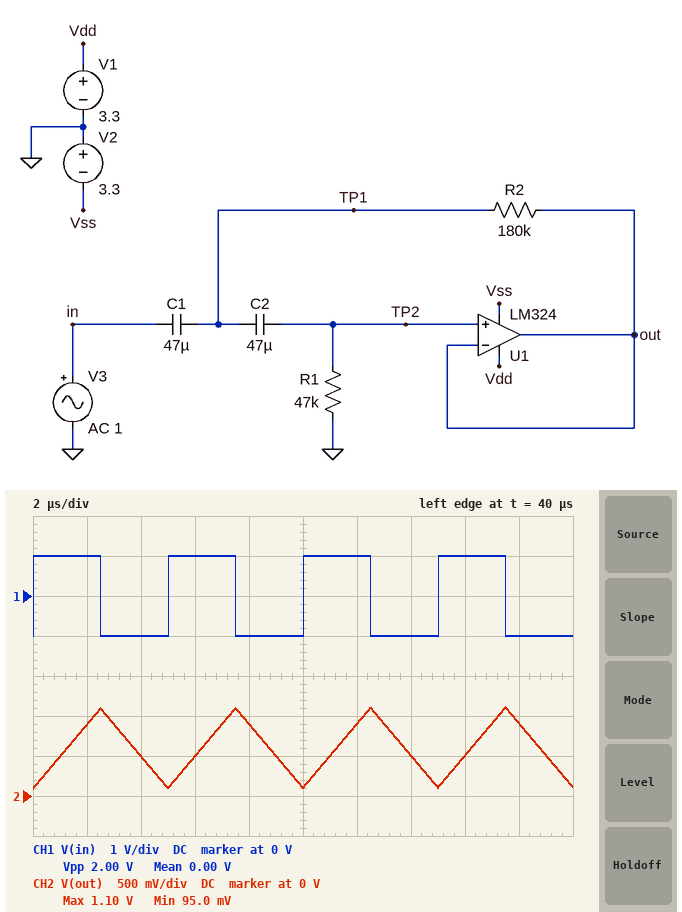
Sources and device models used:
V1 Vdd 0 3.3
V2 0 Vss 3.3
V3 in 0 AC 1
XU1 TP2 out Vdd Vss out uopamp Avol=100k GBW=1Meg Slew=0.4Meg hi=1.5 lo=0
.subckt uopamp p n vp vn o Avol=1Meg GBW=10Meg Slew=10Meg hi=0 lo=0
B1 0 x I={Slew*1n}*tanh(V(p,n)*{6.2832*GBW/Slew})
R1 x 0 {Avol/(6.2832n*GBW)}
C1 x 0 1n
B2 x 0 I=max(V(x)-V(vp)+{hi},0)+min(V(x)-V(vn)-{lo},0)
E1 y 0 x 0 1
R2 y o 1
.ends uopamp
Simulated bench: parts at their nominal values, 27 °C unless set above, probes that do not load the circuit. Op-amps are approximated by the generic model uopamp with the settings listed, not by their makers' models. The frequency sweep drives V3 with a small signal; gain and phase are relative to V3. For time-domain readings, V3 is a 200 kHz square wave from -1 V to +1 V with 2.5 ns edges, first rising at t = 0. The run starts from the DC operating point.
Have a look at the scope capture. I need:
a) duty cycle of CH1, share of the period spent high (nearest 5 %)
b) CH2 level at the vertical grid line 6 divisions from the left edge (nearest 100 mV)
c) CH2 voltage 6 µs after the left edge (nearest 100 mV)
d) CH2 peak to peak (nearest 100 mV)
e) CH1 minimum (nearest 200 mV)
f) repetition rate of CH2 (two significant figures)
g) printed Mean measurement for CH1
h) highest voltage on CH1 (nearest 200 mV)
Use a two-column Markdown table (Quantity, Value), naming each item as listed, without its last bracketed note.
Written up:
| Quantity | Value |
|---|---|
| duty cycle of CH1, share of the period spent high | 50 % |
| CH2 level at the vertical grid line 6 divisions from the left edge | 900 mV |
| CH2 voltage 6 µs after the left edge | 500 mV |
| CH2 peak to peak | 1.0 V |
| CH1 minimum | -1.0 V |
| repetition rate of CH2 | 200 kHz |
| printed Mean measurement for CH1 | 0.00 V |
| highest voltage on CH1 | 1.0 V |
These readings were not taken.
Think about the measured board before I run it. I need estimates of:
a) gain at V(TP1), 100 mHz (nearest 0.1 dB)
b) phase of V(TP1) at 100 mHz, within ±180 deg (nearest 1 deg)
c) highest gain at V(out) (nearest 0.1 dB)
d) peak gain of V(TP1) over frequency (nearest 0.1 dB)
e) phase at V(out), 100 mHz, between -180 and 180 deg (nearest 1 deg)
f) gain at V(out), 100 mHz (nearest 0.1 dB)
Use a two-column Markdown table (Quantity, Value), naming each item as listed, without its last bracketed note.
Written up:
| Quantity | Value |
|---|---|
| gain at V(TP1), 100 mHz | -2.7 dB |
| phase of V(TP1) at 100 mHz, within ±180 deg | 23 deg |
| highest gain at V(out) | 0 dB |
| peak gain of V(TP1) over frequency | 0 dB |
| phase at V(out), 100 mHz, between -180 and 180 deg | 59 deg |
| gain at V(out), 100 mHz | -4.5 dB |
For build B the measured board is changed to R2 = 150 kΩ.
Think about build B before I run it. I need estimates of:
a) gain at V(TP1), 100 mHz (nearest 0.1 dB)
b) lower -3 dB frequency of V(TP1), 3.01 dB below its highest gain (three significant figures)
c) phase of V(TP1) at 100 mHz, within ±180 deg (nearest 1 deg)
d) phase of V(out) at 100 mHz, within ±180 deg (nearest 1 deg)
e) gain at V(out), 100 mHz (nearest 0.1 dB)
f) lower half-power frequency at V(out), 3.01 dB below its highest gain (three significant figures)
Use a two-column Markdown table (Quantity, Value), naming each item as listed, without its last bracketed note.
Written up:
| Quantity | Value |
|---|---|
| gain at V(TP1), 100 mHz | -2.6 dB |
| lower -3 dB frequency of V(TP1), 3.01 dB below its highest gain | 86.5 mHz |
| phase of V(TP1) at 100 mHz, within ±180 deg | 24 deg |
| phase of V(out) at 100 mHz, within ±180 deg | 60 deg |
| gain at V(out), 100 mHz | -4.4 dB |
| lower half-power frequency at V(out), 3.01 dB below its highest gain | 133 mHz |
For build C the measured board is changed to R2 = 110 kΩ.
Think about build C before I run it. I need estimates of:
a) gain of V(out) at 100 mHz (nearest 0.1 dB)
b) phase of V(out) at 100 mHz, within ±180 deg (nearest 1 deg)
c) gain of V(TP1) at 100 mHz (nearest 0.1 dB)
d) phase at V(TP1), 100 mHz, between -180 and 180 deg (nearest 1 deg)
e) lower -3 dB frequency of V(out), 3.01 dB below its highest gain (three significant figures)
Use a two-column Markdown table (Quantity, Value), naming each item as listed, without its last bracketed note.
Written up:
| Quantity | Value |
|---|---|
| gain of V(out) at 100 mHz | -4.3 dB |
| phase of V(out) at 100 mHz, within ±180 deg | 62 deg |
| gain of V(TP1) at 100 mHz | -2.5 dB |
| phase at V(TP1), 100 mHz, between -180 and 180 deg | 26 deg |
| lower -3 dB frequency of V(out), 3.01 dB below its highest gain | 129 mHz |
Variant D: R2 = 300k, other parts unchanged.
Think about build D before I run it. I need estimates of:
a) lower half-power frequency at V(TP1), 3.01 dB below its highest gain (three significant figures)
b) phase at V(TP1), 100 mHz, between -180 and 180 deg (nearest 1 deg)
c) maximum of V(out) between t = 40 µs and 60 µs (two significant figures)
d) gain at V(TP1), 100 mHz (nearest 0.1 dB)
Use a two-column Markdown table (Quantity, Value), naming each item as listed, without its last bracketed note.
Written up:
| Quantity | Value |
|---|---|
| lower half-power frequency at V(TP1), 3.01 dB below its highest gain | 94.0 mHz |
| phase at V(TP1), 100 mHz, between -180 and 180 deg | 22 deg |
| maximum of V(out) between t = 40 µs and 60 µs | 1.1 V |
| gain at V(TP1), 100 mHz | -2.8 dB |
